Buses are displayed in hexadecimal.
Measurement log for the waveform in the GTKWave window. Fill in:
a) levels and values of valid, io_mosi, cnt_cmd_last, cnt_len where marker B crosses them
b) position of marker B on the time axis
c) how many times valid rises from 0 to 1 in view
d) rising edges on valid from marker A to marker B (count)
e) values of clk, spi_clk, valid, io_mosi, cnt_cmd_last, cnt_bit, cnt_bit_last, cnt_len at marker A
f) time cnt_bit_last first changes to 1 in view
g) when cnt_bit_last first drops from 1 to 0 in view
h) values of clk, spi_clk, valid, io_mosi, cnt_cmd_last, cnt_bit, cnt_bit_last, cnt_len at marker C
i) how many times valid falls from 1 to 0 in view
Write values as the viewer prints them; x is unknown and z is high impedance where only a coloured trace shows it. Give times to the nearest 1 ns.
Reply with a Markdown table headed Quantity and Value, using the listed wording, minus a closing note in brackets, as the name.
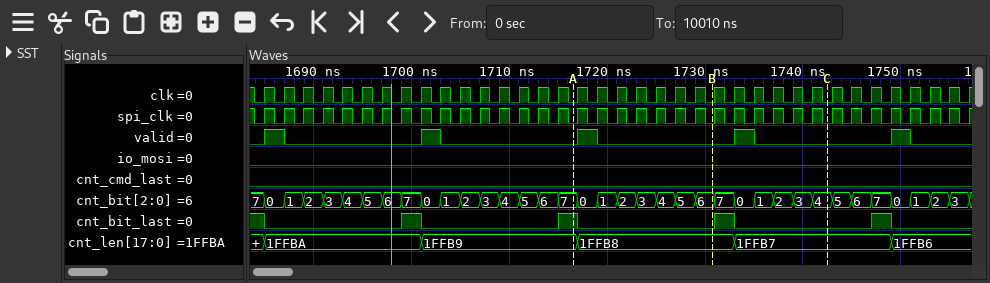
| Quantity | Value |
|---|---|
| levels and values of valid, io_mosi, cnt_cmd_last, cnt_len where marker B crosses them | valid=0, io_mosi=0, cnt_cmd_last=0, cnt_len=1FFB8 |
| position of marker B on the time axis | 1731 ns |
| how many times valid rises from 0 to 1 in view | 5 |
| rising edges on valid from marker A to marker B | 1 |
| values of clk, spi_clk, valid, io_mosi, cnt_cmd_last, cnt_bit, cnt_bit_last, cnt_len at marker A | clk=0, spi_clk=0, valid=0, io_mosi=0, cnt_cmd_last=0, cnt_bit=7, cnt_bit_last=1, cnt_len=1FFB9 |
| time cnt_bit_last first changes to 1 in view | 1699 ns |
| when cnt_bit_last first drops from 1 to 0 in view | 1685 ns |
| values of clk, spi_clk, valid, io_mosi, cnt_cmd_last, cnt_bit, cnt_bit_last, cnt_len at marker C | clk=0, spi_clk=0, valid=0, io_mosi=0, cnt_cmd_last=0, cnt_bit=4, cnt_bit_last=0, cnt_len=1FFB7 |
| how many times valid falls from 1 to 0 in view | 5 |
